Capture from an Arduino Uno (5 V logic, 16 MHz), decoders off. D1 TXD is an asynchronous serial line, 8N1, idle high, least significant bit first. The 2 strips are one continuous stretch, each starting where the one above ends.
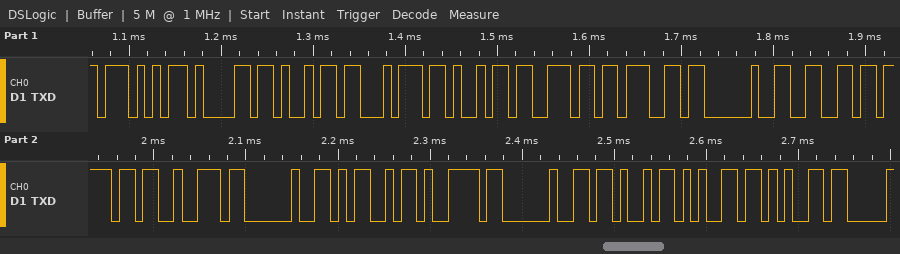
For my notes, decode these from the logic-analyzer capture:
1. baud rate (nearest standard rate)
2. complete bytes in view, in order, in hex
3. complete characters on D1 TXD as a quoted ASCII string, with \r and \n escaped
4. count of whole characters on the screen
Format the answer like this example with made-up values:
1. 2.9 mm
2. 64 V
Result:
1. 115200 baud
2. 0x57 0x61 0x69 0x74 0x69 0x6E 0x67 0x20 0x66 0x6F 0x72 0x20 0x4D 0x79 0x20 0x4B 0x65 0x65
3. "Waiting for My Kee"
4. 18
